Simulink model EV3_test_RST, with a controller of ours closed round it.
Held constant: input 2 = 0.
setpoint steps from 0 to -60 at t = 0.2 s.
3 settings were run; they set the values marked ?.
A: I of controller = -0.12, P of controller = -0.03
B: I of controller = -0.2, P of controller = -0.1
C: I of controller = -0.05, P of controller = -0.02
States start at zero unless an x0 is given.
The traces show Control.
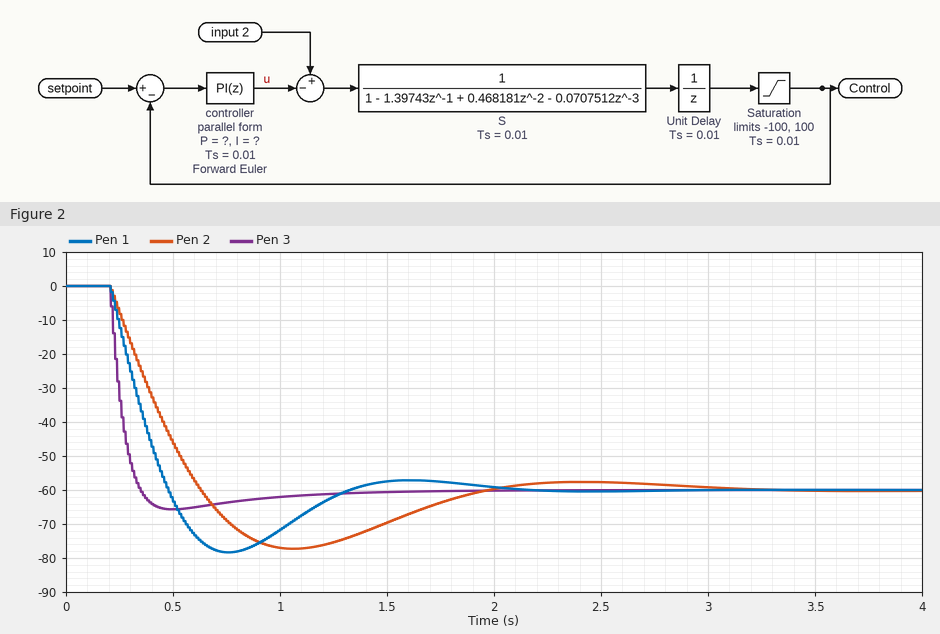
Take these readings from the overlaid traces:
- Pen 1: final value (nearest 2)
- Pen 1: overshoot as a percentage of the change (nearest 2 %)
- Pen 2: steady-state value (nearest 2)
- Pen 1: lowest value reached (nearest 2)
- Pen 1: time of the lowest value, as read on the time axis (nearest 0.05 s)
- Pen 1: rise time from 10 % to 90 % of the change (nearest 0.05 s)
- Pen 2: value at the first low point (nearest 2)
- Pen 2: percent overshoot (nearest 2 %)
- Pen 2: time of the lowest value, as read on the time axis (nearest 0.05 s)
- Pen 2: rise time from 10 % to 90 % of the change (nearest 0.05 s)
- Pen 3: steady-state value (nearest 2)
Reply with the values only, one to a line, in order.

-60
30 %
-60
-78
0.75 s
0.20 s
-78
28 %
1.05 s
0.35 s
-60
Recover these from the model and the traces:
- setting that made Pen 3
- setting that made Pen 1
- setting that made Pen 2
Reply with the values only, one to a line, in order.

B
A
C
